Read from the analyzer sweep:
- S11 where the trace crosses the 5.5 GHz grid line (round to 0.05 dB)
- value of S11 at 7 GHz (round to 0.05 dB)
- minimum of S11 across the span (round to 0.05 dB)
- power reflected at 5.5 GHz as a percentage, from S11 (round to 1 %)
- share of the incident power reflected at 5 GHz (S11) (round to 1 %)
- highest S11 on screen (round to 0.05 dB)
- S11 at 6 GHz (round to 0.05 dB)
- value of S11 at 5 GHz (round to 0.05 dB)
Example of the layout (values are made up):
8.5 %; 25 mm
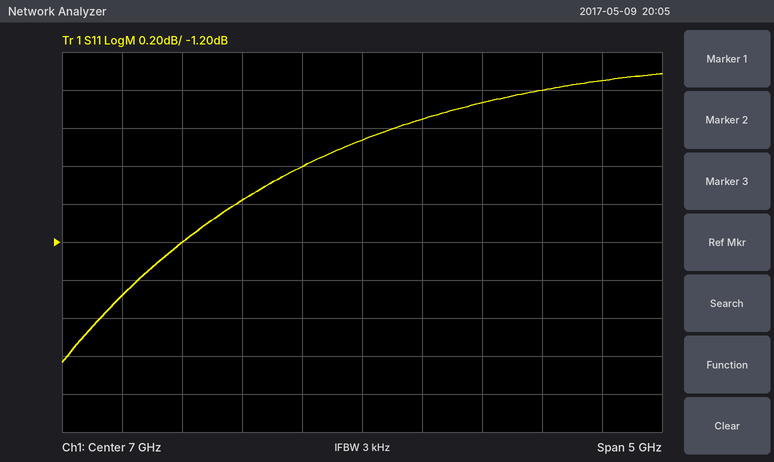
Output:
-1.20 dB; -0.65 dB; -1.85 dB; 76 %; 71 %; -0.30 dB; -1.00 dB; -1.50 dB
